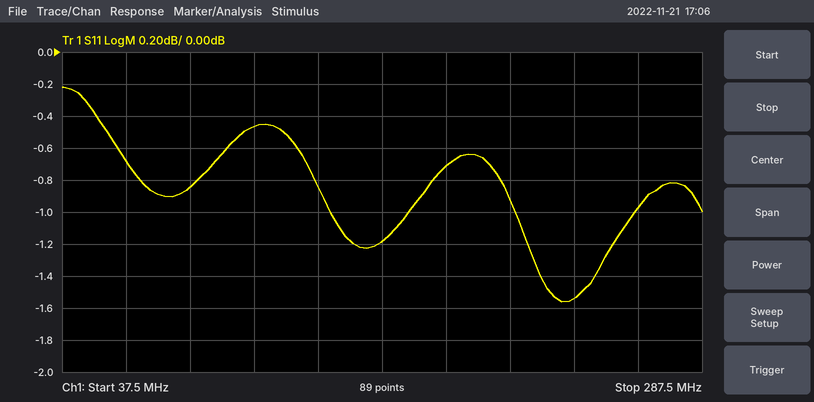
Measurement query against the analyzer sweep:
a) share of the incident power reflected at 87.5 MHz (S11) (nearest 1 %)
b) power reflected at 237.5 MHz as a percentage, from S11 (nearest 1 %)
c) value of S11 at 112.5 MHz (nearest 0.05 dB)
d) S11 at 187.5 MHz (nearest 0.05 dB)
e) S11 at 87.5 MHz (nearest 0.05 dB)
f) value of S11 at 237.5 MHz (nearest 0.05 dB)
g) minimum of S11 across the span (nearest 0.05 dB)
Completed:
82 %
70 %
-0.45 dB
-0.70 dB
-0.85 dB
-1.55 dB
-1.55 dB
